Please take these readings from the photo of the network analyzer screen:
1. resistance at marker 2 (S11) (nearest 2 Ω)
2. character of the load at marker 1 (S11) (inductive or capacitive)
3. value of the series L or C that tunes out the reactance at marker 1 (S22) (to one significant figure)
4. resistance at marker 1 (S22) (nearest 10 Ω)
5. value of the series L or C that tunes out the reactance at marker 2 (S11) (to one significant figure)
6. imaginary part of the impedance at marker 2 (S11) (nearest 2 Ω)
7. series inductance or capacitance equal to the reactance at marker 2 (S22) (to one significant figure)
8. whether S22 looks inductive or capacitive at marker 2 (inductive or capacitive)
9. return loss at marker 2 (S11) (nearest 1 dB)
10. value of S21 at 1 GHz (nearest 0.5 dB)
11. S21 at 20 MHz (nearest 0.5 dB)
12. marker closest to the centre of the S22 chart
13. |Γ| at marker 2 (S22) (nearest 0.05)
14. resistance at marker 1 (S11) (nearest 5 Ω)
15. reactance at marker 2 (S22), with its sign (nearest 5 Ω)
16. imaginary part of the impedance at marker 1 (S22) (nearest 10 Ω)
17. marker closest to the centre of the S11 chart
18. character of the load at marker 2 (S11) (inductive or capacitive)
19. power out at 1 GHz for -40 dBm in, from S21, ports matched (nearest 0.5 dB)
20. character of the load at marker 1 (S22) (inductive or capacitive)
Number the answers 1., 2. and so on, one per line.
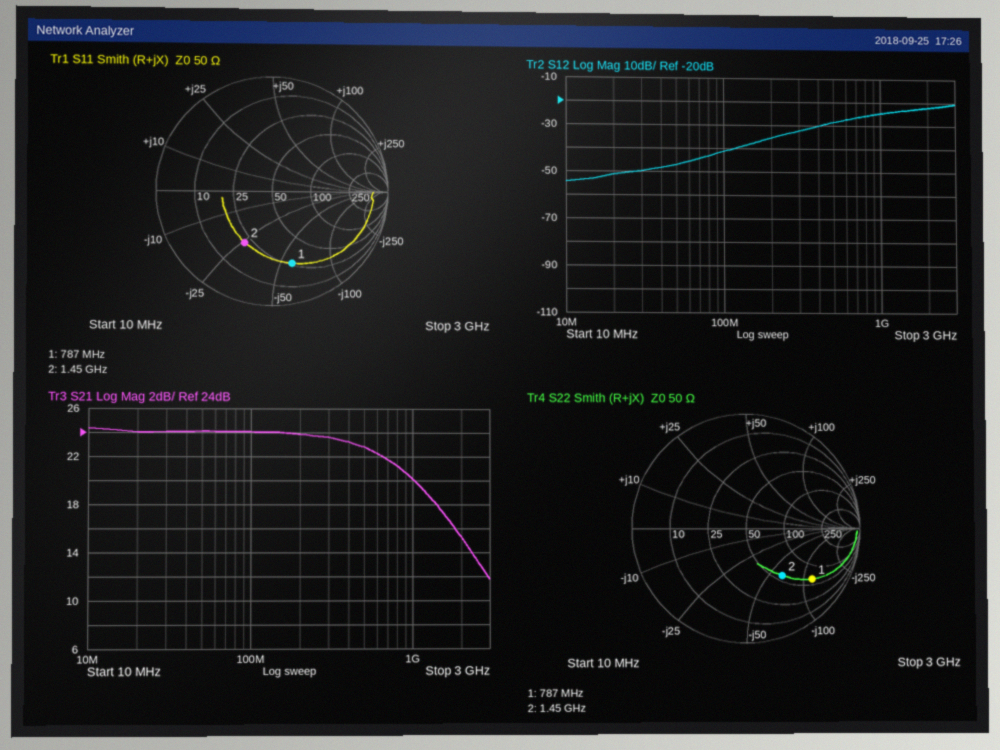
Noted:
1. 22 Ω
2. capacitive
3. 20 nH
4. 60 Ω
5. 3 nH
6. -26 Ω
7. 2 pF
8. capacitive
9. 6 dB
10. 20.0 dB
11. 24.0 dB
12. marker 2
13. 0.50
14. 25 Ω
15. -65 Ω
16. -120 Ω
17. marker 2
18. capacitive
19. -20.0 dBm
20. capacitive
